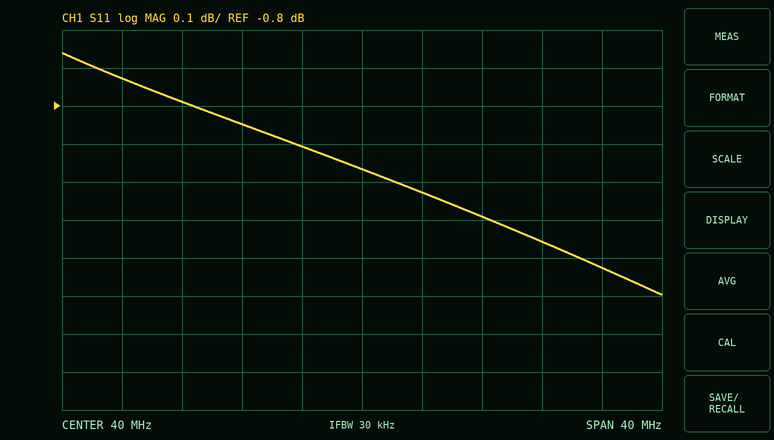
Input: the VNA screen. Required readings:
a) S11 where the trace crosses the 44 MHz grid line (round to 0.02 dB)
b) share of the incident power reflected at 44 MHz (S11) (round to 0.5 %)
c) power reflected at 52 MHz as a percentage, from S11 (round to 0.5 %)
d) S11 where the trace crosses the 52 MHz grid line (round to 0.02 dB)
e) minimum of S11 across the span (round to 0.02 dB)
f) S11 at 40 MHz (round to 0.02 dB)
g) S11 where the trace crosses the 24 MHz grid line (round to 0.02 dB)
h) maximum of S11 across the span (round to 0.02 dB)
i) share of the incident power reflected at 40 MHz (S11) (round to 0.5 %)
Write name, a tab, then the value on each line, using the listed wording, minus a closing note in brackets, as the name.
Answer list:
S11 where the trace crosses the 44 MHz grid line	-1.02 dB
share of the incident power reflected at 44 MHz (S11)	79.0 %
power reflected at 52 MHz as a percentage, from S11	76.5 %
S11 where the trace crosses the 52 MHz grid line	-1.16 dB
minimum of S11 across the span	-1.30 dB
S11 at 40 MHz	-0.96 dB
S11 where the trace crosses the 24 MHz grid line	-0.72 dB
maximum of S11 across the span	-0.66 dB
share of the incident power reflected at 40 MHz (S11)	80.0 %
